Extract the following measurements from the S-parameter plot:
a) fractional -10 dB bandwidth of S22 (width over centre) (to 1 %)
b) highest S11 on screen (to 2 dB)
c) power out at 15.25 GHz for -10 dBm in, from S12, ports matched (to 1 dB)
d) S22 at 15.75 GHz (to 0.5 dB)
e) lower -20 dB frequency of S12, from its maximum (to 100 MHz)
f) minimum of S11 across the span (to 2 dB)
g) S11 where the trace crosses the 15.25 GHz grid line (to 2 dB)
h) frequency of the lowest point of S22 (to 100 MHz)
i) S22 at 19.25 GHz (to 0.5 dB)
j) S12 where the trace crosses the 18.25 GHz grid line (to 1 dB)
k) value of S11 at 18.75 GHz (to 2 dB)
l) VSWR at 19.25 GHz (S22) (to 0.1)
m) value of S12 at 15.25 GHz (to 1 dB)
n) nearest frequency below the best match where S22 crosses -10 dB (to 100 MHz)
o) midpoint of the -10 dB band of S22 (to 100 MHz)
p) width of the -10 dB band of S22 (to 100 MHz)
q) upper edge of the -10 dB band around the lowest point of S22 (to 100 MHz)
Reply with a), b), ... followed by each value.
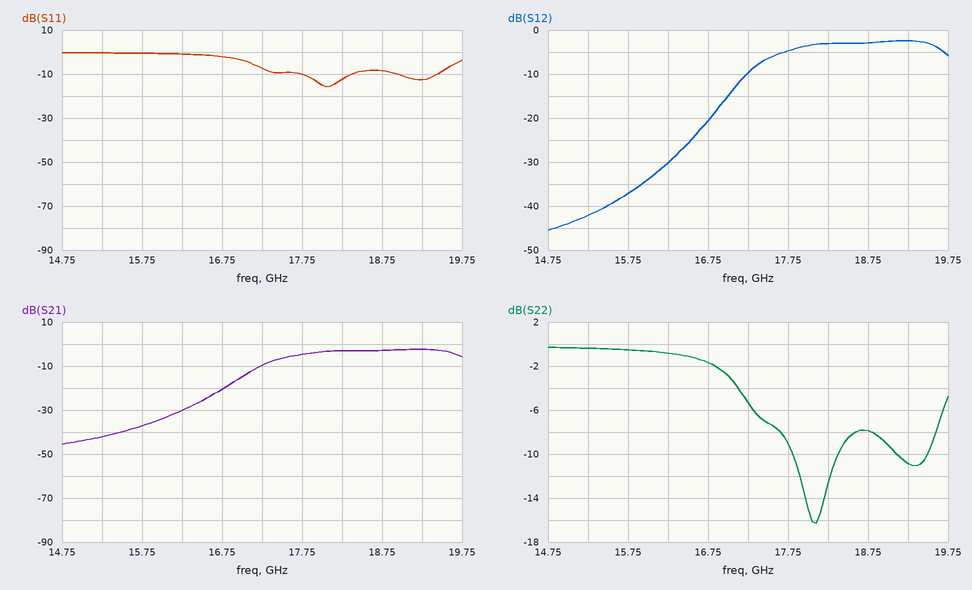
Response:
a) 3 %
b) 0 dB
c) -52 dBm
d) -0.5 dB
e) 16.7 GHz
f) -16 dB
g) 0 dB
h) 18.1 GHz
i) -11.0 dB
j) -3 dB
k) -8 dB
l) 1.8
m) -42 dB
n) 17.8 GHz
o) 18.1 GHz
p) 600 MHz
q) 18.4 GHz
